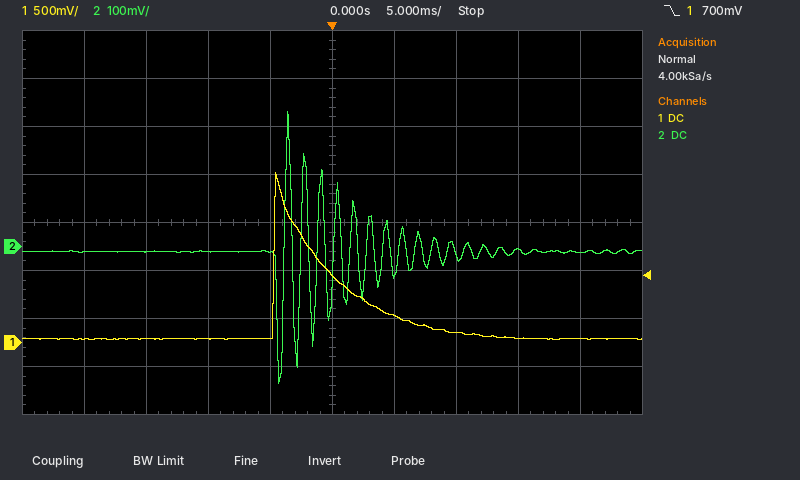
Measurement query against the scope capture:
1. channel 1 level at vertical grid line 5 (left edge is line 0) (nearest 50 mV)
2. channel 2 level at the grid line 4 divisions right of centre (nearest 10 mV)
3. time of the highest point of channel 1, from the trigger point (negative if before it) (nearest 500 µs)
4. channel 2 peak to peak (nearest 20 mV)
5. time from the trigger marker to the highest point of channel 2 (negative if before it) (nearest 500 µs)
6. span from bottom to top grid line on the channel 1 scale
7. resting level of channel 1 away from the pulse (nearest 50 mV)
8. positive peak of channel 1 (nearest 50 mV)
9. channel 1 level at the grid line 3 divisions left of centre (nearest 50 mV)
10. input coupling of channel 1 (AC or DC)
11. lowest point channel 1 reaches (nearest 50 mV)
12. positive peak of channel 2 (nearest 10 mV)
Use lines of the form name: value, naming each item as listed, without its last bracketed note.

channel 1 level at vertical grid line 5 (left edge is line 0): 700 mV
channel 2 level at the grid line 4 divisions right of centre: -10 mV
time of the highest point of channel 1, from the trigger point (negative if before it): -4.5 ms
channel 2 peak to peak: 560 mV
time from the trigger marker to the highest point of channel 2 (negative if before it): -3.5 ms
span from bottom to top grid line on the channel 1 scale: 4 V
resting level of channel 1 away from the pulse: 50 mV
positive peak of channel 1: 1.75 V
channel 1 level at the grid line 3 divisions left of centre: 50 mV
input coupling of channel 1: DC
lowest point channel 1 reaches: 50 mV
positive peak of channel 2: 280 mV
